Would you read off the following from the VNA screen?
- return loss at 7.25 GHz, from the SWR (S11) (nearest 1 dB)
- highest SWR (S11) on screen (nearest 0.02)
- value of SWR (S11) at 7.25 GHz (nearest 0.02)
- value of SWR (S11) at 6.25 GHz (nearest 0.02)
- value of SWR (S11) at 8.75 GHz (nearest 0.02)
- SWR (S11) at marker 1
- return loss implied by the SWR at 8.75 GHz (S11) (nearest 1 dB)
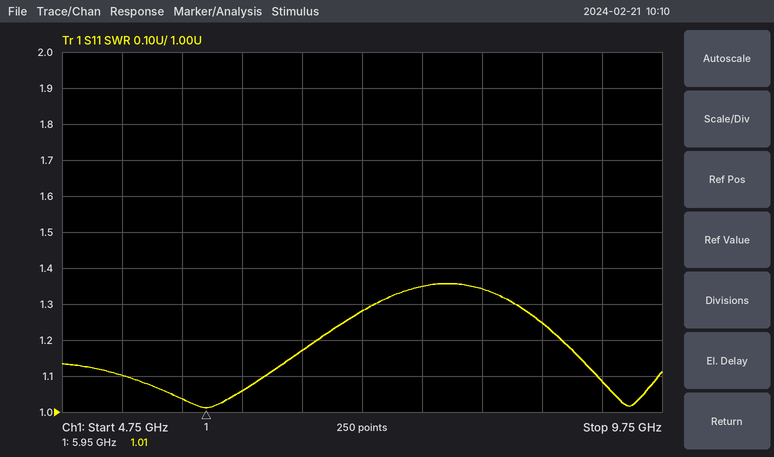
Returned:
18 dB
1.36
1.28
1.06
1.24
1.01
19 dB
